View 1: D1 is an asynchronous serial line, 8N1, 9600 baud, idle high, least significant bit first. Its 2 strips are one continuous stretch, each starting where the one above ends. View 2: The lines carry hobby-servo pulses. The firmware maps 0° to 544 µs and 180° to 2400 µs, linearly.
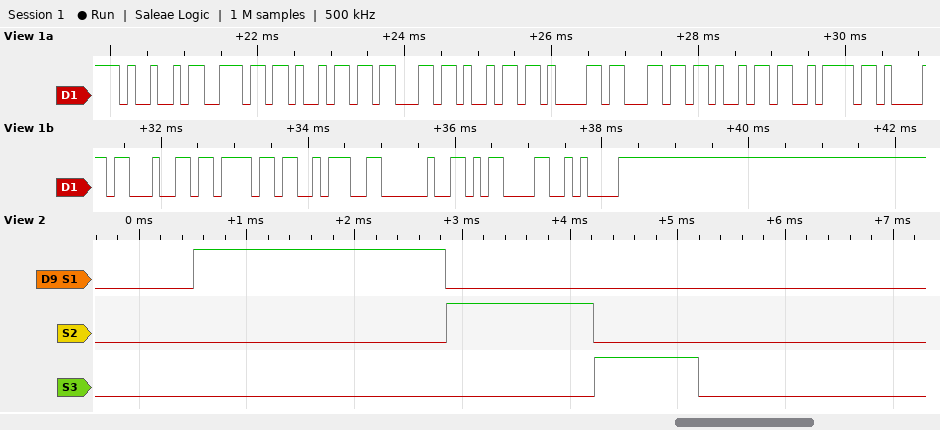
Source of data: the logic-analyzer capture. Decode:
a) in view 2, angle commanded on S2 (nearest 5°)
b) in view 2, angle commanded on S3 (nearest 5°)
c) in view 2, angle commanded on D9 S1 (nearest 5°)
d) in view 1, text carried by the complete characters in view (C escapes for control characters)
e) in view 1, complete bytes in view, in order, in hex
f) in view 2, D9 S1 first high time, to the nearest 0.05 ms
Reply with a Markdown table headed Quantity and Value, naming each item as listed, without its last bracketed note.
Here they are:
| Quantity | Value |
|---|---|
| in view 2, angle commanded on S2 | 80° |
| in view 2, angle commanded on S3 | 40° |
| in view 2, angle commanded on D9 S1 | 175° |
| in view 1, text carried by the complete characters in view | "Inicializado: \r\n" |
| in view 1, complete bytes in view, in order, in hex | 49 6E 69 63 69 61 6C 69 7A 61 64 6F 3A 20 0D 0A |
| in view 2, D9 S1 first high time, to the nearest 0.05 ms | 2.35 ms |
